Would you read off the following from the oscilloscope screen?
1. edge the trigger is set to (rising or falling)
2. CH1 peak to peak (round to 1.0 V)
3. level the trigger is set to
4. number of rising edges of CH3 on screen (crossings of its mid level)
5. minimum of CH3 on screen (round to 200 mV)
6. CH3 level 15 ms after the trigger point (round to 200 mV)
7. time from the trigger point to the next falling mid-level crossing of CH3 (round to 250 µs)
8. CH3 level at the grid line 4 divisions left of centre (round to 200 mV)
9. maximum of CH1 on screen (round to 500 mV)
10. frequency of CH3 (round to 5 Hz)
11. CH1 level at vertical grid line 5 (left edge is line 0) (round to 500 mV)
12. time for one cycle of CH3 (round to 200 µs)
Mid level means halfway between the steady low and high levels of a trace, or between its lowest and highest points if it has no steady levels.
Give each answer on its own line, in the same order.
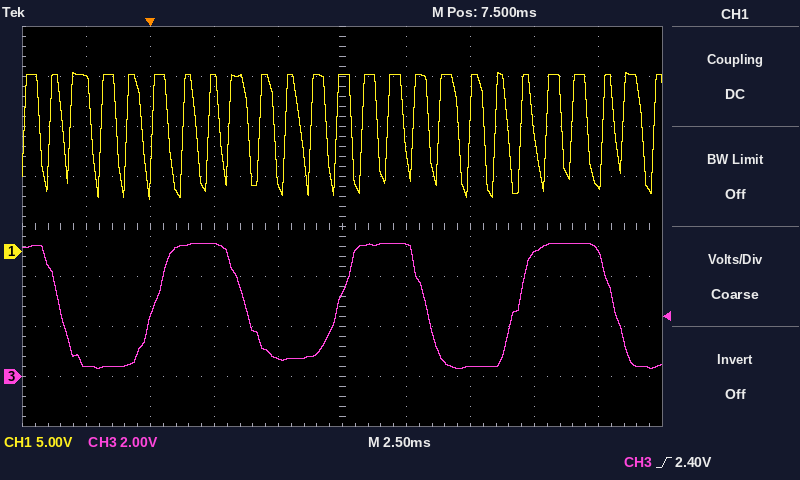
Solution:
rising
13.0 V
2.40 V
3
400 mV
5.0 V
3.75 ms
400 mV
18.0 V
140 Hz
17.5 V
7.2 ms
